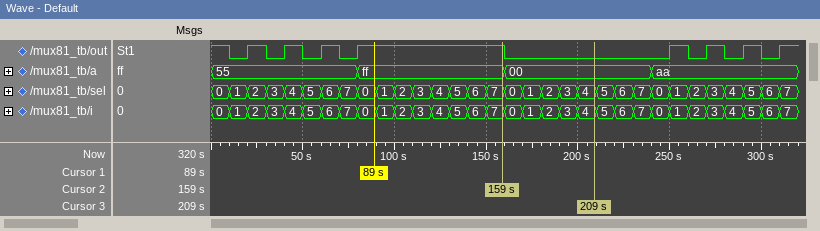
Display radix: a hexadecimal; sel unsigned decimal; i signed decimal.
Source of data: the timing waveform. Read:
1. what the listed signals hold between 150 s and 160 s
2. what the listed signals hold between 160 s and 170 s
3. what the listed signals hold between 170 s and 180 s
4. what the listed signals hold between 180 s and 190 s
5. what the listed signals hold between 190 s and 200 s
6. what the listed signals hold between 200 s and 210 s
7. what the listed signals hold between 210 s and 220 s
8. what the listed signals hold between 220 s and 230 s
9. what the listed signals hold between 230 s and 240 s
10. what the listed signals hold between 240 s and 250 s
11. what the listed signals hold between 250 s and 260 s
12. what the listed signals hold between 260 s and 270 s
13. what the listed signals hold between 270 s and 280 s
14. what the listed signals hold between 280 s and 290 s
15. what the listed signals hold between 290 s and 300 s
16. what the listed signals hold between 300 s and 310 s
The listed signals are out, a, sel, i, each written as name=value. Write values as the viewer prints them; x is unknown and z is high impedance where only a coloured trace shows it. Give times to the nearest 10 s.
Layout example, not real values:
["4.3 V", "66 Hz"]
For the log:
["out=1, a=ff, sel=7, i=7", "out=0, a=00, sel=0, i=0", "out=0, a=00, sel=1, i=1", "out=0, a=00, sel=2, i=2", "out=0, a=00, sel=3, i=3", "out=0, a=00, sel=4, i=4", "out=0, a=00, sel=5, i=5", "out=0, a=00, sel=6, i=6", "out=0, a=00, sel=7, i=7", "out=0, a=aa, sel=0, i=0", "out=1, a=aa, sel=1, i=1", "out=0, a=aa, sel=2, i=2", "out=1, a=aa, sel=3, i=3", "out=0, a=aa, sel=4, i=4", "out=1, a=aa, sel=5, i=5", "out=0, a=aa, sel=6, i=6"]
